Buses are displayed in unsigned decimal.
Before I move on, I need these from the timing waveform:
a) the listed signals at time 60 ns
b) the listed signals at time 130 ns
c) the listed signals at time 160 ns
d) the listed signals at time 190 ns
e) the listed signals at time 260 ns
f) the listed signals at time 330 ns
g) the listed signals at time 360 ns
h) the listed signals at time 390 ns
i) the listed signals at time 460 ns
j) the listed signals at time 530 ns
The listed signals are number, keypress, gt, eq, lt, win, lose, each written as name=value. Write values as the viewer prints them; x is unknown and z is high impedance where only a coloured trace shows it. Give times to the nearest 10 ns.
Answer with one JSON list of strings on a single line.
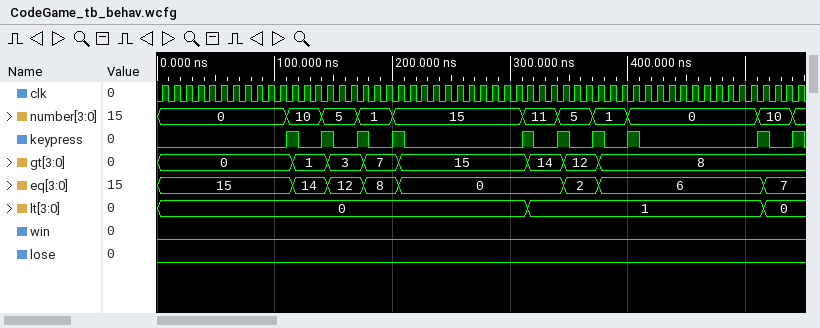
["number=0, keypress=0, gt=0, eq=15, lt=0, win=0, lose=0", "number=10, keypress=0, gt=1, eq=14, lt=0, win=0, lose=0", "number=5, keypress=0, gt=3, eq=12, lt=0, win=0, lose=0", "number=1, keypress=0, gt=7, eq=8, lt=0, win=0, lose=0", "number=15, keypress=0, gt=15, eq=0, lt=0, win=0, lose=0", "number=11, keypress=0, gt=14, eq=0, lt=1, win=0, lose=0", "number=5, keypress=0, gt=12, eq=2, lt=1, win=0, lose=0", "number=1, keypress=0, gt=8, eq=6, lt=1, win=0, lose=0", "number=0, keypress=0, gt=8, eq=6, lt=1, win=0, lose=0", "number=10, keypress=0, gt=8, eq=7, lt=0, win=0, lose=0"]
